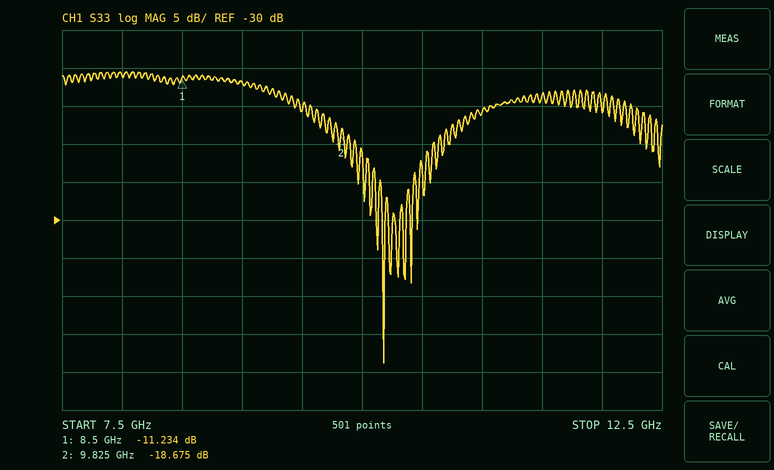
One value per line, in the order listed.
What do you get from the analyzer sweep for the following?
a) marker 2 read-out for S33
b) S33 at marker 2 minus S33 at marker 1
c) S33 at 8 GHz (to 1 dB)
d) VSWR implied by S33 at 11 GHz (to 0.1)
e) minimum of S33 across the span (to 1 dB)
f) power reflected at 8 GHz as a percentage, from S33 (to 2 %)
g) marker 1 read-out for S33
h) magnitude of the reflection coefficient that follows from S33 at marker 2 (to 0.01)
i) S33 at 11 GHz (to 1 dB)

-18.675 dB
-7.441 dB
-11 dB
1.4
-49 dB
8 %
-11.234 dB
0.12
-16 dB
